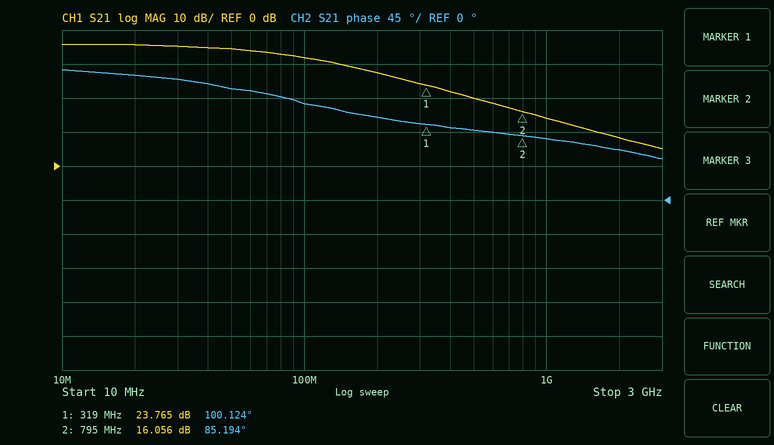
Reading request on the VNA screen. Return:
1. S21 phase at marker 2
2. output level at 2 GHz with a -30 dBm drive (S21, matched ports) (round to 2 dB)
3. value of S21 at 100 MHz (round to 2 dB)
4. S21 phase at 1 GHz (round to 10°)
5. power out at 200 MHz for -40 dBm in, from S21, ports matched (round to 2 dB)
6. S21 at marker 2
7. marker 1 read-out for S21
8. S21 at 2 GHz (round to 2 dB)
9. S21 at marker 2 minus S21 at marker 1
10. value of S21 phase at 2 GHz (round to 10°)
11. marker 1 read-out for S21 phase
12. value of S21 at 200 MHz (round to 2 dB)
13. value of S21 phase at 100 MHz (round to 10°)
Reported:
85.194°
-22 dBm
32 dB
80°
-12 dBm
16.056 dB
23.765 dB
8 dB
-7.709 dB
70°
100.124°
28 dB
130°
